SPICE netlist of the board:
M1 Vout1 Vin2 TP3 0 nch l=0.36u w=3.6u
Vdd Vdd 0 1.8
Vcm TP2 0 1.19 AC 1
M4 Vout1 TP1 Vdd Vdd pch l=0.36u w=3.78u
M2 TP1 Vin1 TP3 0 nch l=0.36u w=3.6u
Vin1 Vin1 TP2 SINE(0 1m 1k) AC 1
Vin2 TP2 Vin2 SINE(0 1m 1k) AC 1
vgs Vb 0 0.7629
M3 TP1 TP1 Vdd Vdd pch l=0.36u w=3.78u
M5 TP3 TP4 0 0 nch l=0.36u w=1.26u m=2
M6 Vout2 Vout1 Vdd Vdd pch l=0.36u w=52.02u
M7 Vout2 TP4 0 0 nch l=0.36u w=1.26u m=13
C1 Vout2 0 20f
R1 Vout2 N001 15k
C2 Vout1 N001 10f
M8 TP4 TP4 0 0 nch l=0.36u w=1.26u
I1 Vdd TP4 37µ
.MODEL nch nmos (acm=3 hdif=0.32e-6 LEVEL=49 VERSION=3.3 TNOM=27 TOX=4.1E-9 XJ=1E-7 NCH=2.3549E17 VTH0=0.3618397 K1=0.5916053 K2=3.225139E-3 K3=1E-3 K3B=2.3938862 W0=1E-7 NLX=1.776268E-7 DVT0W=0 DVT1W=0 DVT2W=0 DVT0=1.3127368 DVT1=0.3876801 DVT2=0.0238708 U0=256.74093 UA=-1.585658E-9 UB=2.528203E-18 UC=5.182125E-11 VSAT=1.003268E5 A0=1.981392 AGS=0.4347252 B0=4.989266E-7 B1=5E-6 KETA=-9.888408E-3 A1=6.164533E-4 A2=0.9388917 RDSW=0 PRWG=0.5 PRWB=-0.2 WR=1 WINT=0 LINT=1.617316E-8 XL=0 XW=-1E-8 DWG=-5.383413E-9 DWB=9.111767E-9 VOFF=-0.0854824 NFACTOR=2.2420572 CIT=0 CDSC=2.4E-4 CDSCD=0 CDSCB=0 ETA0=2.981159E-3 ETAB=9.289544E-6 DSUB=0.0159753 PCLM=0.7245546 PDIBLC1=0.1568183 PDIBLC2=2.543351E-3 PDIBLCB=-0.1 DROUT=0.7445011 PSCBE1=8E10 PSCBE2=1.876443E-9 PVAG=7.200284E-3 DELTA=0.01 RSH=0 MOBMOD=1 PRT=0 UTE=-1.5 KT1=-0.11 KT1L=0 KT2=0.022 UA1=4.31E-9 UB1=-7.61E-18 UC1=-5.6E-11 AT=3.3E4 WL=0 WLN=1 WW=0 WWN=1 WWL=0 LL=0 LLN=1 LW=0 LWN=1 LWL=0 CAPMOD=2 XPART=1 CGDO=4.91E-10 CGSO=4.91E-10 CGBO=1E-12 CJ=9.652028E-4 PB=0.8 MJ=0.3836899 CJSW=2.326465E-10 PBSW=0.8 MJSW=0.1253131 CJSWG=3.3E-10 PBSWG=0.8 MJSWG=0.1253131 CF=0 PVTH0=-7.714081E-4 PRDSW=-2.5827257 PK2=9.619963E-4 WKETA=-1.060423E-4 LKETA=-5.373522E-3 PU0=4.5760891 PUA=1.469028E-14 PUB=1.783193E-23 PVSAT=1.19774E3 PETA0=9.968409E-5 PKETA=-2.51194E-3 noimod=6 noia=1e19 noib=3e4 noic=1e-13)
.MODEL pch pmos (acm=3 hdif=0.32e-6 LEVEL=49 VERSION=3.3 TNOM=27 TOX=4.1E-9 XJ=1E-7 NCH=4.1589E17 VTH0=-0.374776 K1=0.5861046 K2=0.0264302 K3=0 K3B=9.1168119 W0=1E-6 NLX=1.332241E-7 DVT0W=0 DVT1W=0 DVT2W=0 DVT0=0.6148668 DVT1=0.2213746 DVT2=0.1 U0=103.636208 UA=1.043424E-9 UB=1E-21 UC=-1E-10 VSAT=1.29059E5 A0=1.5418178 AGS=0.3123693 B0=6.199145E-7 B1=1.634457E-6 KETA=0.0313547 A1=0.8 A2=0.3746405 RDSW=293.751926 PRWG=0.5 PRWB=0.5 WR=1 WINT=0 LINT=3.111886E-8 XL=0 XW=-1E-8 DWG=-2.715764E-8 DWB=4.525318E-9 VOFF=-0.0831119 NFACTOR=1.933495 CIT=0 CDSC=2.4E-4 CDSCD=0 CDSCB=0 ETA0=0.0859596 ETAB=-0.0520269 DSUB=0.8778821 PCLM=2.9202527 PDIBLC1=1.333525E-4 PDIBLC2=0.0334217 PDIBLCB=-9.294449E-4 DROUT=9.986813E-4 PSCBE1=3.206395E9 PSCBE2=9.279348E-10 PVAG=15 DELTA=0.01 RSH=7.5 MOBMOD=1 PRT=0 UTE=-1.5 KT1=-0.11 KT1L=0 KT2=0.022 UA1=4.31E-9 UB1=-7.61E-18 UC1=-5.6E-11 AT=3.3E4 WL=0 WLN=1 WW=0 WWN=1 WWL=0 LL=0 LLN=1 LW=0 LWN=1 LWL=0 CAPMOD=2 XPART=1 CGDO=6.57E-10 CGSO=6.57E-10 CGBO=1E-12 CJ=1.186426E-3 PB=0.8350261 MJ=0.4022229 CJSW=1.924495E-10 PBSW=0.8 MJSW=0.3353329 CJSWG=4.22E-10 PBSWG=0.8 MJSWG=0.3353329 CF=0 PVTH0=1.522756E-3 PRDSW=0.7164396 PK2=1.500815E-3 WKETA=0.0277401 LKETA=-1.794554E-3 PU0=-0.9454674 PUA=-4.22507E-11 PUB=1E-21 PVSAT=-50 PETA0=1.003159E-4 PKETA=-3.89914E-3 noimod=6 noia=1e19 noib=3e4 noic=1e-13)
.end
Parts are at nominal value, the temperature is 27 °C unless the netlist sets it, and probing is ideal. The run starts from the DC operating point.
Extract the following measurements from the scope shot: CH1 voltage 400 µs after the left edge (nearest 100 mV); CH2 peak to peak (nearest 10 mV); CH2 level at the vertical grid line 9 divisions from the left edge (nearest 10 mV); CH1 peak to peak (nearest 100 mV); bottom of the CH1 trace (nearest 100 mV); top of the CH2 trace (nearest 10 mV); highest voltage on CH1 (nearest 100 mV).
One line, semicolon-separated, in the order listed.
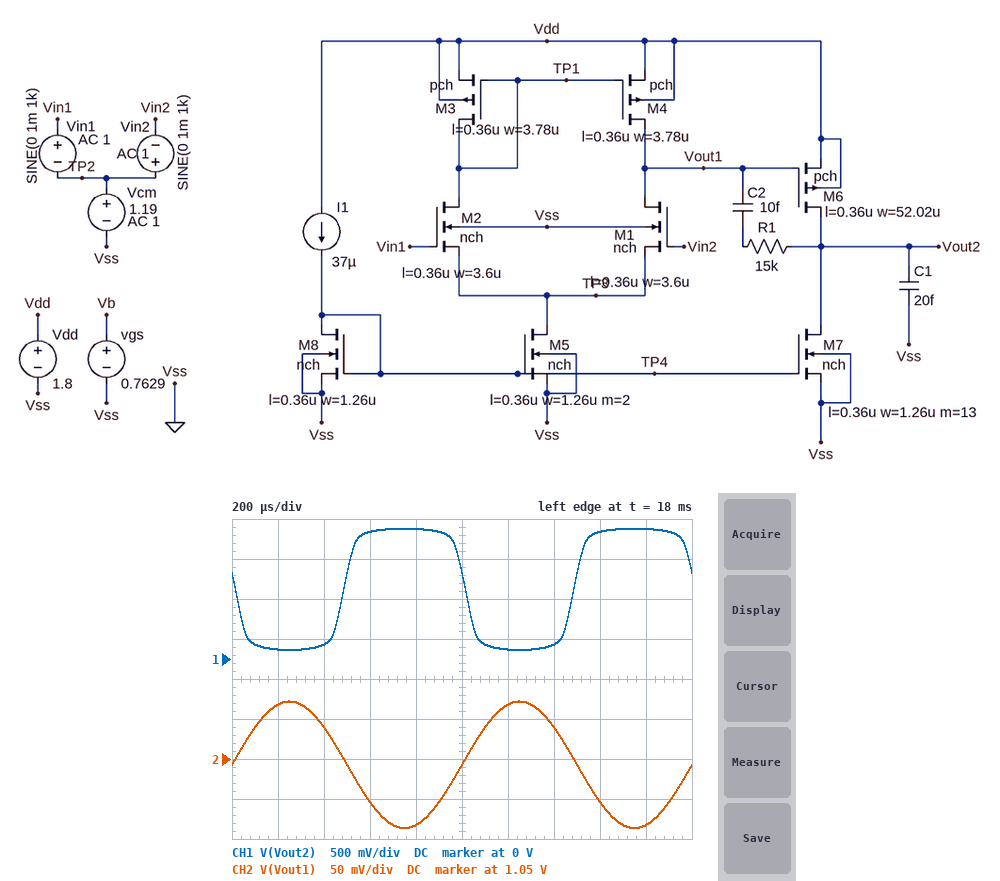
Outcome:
200 mV; 160 mV; 970 mV; 1.5 V; 100 mV; 1.12 V; 1.6 V
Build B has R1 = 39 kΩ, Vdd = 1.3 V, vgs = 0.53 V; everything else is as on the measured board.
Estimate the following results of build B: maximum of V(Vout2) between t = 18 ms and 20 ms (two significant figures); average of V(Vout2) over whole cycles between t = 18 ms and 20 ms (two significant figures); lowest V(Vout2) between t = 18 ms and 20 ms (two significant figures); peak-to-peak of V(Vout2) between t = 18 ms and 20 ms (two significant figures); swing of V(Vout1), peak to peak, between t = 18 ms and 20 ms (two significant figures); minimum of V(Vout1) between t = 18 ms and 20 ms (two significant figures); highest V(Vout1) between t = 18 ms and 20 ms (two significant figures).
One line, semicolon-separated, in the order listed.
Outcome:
840 mV; 750 mV; 650 mV; 190 mV; 8.6 mV; 540 mV; 550 mV
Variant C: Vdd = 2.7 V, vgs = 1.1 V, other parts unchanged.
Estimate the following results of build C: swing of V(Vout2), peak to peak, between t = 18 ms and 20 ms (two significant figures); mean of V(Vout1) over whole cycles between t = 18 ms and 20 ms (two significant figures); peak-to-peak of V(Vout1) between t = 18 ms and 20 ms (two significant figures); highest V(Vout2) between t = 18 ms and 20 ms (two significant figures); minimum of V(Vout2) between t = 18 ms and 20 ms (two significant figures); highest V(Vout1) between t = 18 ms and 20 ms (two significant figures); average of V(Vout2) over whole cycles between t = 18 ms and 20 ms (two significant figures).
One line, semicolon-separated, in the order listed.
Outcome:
2.4 V; 1.9 V; 170 mV; 2.5 V; 120 mV; 2.0 V; 1.4 V
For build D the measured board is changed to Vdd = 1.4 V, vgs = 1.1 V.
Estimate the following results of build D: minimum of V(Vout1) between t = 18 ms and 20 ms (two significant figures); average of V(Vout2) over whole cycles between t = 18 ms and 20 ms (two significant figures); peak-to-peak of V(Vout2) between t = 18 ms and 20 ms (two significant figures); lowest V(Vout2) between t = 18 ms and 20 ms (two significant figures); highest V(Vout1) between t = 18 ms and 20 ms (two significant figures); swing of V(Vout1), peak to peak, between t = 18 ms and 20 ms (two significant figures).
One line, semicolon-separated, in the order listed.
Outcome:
620 mV; 730 mV; 950 mV; 200 mV; 680 mV; 60 mV
